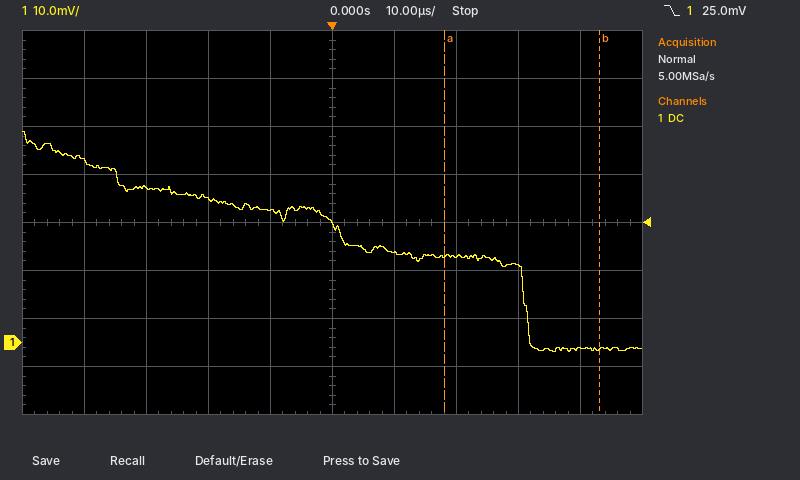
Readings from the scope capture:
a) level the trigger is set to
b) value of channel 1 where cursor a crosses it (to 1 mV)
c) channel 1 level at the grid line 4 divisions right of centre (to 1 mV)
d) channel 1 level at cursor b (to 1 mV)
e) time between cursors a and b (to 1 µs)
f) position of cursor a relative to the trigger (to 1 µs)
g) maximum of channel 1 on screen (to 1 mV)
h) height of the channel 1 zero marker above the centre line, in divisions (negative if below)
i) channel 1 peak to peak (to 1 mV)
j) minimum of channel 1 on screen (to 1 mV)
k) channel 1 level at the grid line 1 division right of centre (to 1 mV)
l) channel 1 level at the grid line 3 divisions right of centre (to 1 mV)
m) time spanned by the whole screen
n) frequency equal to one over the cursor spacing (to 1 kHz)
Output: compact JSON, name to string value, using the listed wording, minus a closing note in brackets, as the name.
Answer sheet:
{"level the trigger is set to": "25.0 mV", "value of channel 1 where cursor a crosses it": "18 mV", "channel 1 level at the grid line 4 divisions right of centre": "-1 mV", "channel 1 level at cursor b": "-1 mV", "time between cursors a and b": "25 µs", "position of cursor a relative to the trigger": "+18 µs", "maximum of channel 1 on screen": "44 mV", "height of the channel 1 zero marker above the centre line, in divisions": "-2.5 div", "channel 1 peak to peak": "46 mV", "minimum of channel 1 on screen": "-2 mV", "channel 1 level at the grid line 1 division right of centre": "19 mV", "channel 1 level at the grid line 3 divisions right of centre": "16 mV", "time spanned by the whole screen": "100 µs", "frequency equal to one over the cursor spacing": "40 kHz"}
